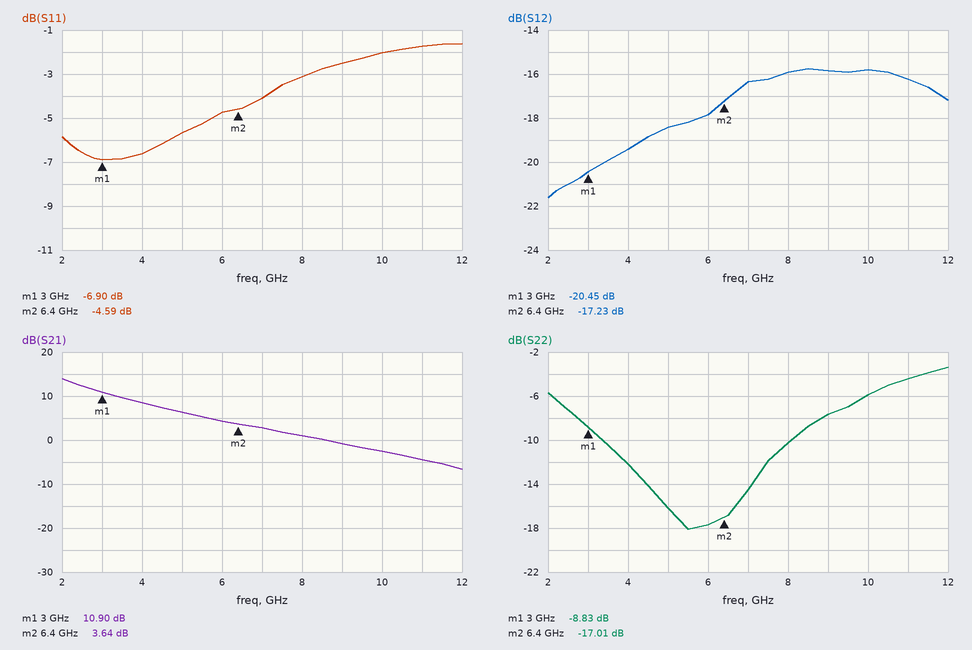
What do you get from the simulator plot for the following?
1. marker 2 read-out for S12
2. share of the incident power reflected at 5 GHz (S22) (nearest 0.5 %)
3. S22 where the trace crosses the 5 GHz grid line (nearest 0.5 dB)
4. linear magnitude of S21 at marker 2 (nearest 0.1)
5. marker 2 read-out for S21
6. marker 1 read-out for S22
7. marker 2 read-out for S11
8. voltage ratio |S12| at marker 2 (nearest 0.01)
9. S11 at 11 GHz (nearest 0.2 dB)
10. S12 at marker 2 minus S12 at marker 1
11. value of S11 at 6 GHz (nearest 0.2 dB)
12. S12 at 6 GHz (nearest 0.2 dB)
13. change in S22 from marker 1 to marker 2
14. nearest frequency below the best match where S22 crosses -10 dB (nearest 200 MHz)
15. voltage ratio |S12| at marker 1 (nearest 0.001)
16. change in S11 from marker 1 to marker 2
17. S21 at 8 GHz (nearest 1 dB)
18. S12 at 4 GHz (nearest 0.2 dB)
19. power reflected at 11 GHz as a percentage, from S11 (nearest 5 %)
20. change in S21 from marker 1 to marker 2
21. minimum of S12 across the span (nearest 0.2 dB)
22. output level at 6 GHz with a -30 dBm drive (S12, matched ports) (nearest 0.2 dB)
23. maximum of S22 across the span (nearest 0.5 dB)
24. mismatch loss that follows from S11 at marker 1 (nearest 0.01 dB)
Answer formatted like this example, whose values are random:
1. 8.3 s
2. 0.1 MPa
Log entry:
1. -17.23 dB
2. 2.5 %
3. -16.0 dB
4. 1.5
5. 3.64 dB
6. -8.83 dB
7. -4.59 dB
8. 0.14
9. -1.8 dB
10. 3.22 dB
11. -4.8 dB
12. -17.8 dB
13. -8.18 dB
14. 3.4 GHz
15. 0.095
16. 2.31 dB
17. 1 dB
18. -19.4 dB
19. 65 %
20. -7.26 dB
21. -21.6 dB
22. -47.8 dBm
23. -3.5 dB
24. 0.99 dB
